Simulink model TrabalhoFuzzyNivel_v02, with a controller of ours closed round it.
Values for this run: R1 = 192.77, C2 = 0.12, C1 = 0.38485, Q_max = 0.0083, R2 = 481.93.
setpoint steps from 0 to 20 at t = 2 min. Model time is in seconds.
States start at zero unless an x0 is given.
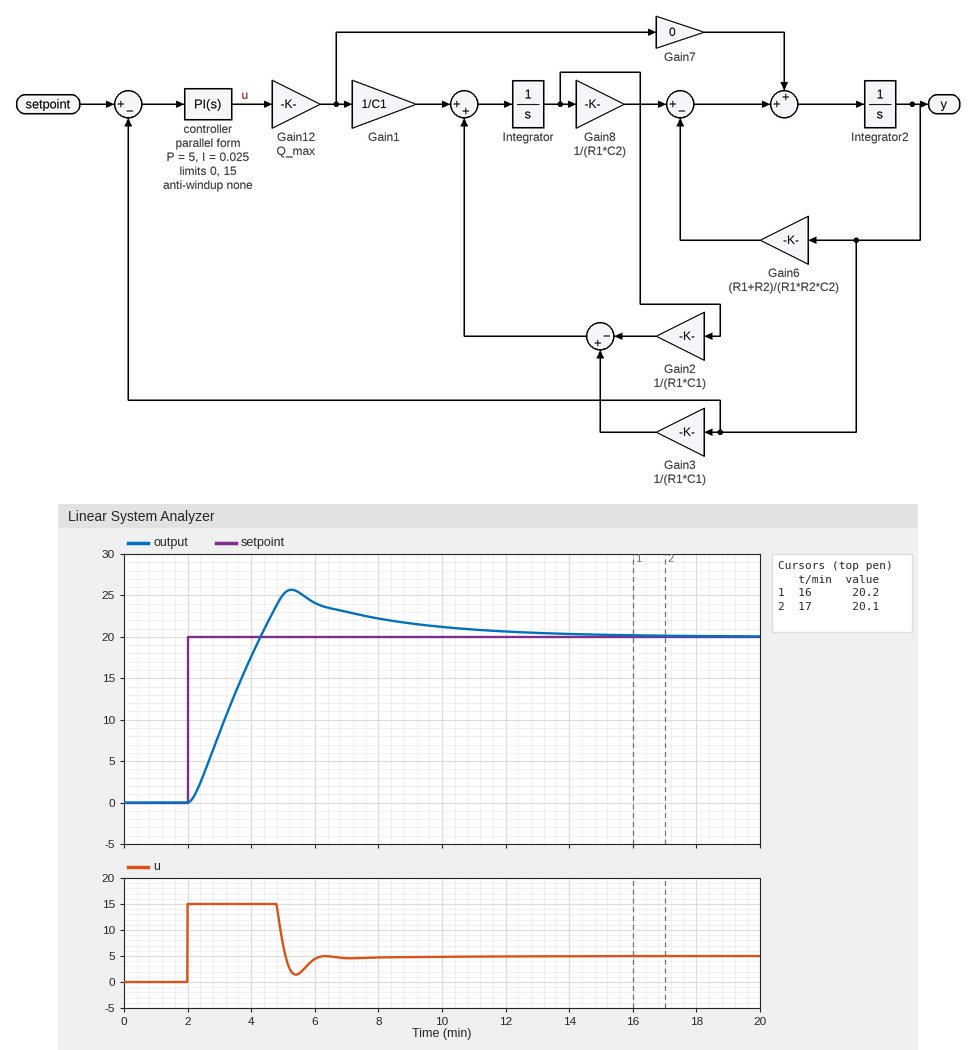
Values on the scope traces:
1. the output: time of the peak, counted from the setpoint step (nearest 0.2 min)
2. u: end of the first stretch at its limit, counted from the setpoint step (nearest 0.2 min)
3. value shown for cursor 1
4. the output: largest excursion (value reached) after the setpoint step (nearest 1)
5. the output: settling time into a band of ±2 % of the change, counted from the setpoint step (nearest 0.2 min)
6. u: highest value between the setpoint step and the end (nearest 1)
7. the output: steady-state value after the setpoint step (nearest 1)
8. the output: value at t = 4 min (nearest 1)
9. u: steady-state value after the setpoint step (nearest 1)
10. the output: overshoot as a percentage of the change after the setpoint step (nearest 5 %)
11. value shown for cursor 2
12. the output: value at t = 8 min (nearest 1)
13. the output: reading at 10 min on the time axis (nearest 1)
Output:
3.2 min
2.8 min
20.2
26
11.6 min
15
20
18
5
30 %
20.1
22
21
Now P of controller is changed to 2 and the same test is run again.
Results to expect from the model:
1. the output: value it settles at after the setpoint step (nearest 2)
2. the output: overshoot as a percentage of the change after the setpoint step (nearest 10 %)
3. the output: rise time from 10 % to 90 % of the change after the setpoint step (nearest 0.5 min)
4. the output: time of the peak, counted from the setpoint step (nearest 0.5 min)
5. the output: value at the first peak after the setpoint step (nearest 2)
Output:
20
50 %
1.5 min
4.0 min
30
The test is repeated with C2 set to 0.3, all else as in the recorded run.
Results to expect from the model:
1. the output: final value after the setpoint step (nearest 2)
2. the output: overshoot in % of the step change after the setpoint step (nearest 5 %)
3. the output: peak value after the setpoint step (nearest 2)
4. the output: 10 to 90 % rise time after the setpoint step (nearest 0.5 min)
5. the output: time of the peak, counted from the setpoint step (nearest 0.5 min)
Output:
20
40 %
28
2.0 min
4.5 min
